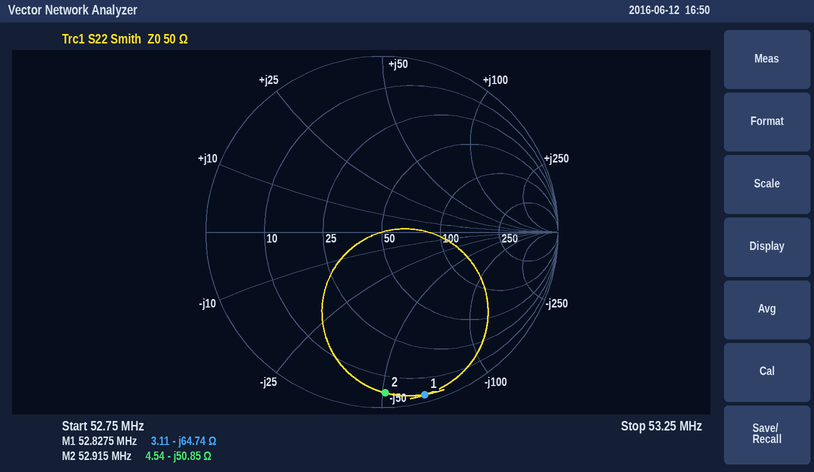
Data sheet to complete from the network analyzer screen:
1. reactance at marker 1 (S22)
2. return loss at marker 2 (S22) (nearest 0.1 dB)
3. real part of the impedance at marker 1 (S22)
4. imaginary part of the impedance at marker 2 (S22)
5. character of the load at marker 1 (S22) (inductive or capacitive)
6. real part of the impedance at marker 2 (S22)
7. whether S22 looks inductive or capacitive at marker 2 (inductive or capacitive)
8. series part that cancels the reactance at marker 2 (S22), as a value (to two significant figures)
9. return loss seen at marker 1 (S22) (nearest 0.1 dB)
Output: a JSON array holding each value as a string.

["-64.74 Ω", "0.8 dB", "3.11 Ω", "-50.85 Ω", "capacitive", "4.54 Ω", "capacitive", "150 nH", "0.4 dB"]
